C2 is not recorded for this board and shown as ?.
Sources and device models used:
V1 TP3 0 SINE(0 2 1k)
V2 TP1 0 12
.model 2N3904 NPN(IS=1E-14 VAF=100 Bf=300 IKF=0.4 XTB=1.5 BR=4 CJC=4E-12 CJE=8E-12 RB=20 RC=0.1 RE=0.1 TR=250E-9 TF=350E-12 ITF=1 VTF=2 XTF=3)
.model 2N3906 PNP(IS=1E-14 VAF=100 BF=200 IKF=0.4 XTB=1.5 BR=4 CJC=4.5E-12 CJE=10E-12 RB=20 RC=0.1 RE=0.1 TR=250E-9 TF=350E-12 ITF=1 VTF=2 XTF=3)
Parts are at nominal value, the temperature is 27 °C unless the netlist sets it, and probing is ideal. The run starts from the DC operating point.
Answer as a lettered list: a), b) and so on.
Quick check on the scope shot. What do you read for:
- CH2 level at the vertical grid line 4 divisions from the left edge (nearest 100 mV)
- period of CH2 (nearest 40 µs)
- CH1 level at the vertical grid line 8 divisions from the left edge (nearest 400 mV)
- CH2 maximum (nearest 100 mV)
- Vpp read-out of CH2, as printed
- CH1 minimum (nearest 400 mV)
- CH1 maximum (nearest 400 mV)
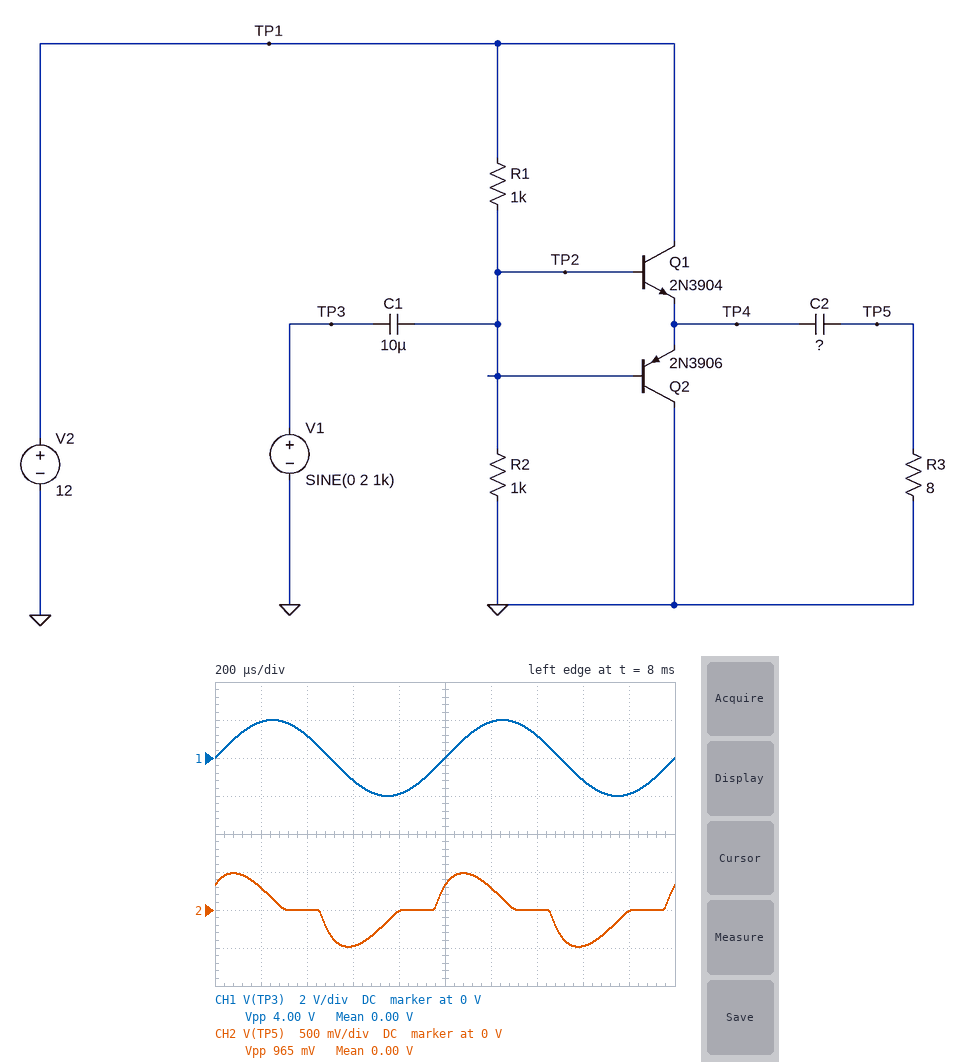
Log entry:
a) 0 V
b) 1.00 ms
c) -1.2 V
d) 500 mV
e) 965 mV
f) -2.0 V
g) 2.0 V
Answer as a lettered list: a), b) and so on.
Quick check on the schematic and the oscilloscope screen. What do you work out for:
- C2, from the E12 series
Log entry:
a) 5.6 µF
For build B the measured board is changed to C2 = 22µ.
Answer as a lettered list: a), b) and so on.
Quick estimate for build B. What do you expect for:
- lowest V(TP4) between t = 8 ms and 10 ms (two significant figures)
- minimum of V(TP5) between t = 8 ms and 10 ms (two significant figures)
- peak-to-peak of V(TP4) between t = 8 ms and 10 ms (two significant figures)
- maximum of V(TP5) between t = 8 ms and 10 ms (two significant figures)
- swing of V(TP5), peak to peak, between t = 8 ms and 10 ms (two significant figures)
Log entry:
a) 4.8 V
b) -1.0 V
c) 2.4 V
d) 1.0 V
e) 2.0 V
